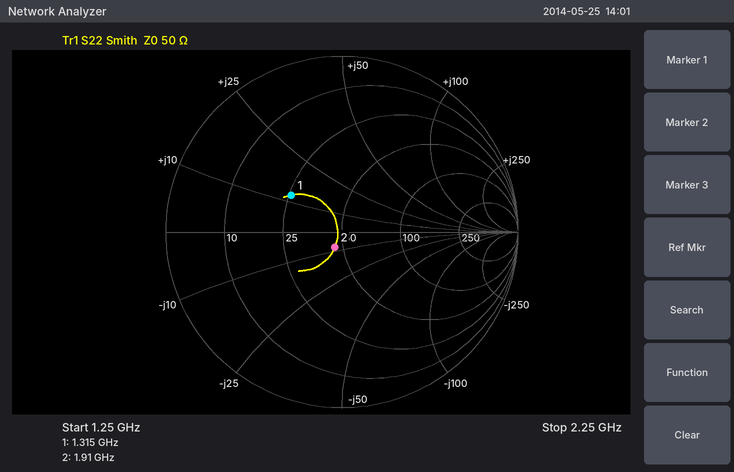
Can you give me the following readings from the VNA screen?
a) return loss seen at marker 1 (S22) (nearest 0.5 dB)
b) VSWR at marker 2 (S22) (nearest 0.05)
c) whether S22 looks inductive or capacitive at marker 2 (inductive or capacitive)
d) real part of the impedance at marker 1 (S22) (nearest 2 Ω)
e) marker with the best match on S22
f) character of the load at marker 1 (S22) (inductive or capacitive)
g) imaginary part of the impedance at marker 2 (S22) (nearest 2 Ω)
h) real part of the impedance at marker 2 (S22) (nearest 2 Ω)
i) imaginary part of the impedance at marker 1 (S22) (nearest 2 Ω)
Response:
9.0 dB
1.20
capacitive
26 Ω
marker 2
inductive
-8 Ω
46 Ω
+12 Ω
